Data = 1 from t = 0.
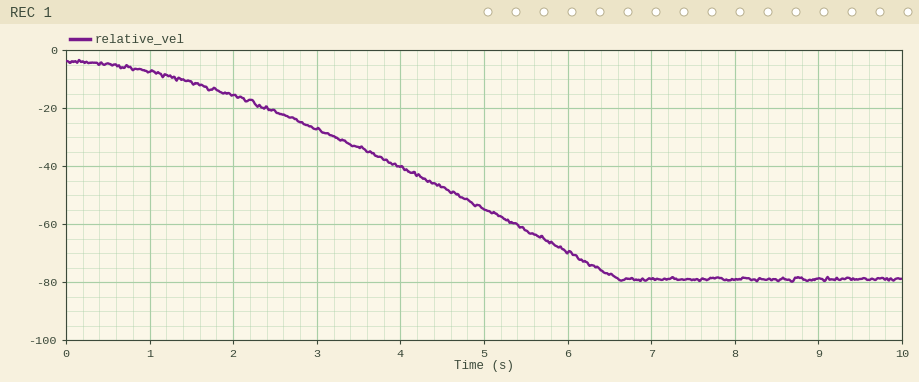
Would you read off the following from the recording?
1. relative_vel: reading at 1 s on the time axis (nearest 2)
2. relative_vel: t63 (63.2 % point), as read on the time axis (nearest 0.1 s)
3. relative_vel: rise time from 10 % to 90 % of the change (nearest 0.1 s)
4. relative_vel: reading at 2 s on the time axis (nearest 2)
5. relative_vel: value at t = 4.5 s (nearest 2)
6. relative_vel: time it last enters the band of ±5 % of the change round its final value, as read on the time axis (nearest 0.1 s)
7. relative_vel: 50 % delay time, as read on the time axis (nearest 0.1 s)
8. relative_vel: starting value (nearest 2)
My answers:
-8
4.8 s
4.6 s
-16
-48
6.4 s
4.1 s
-4
